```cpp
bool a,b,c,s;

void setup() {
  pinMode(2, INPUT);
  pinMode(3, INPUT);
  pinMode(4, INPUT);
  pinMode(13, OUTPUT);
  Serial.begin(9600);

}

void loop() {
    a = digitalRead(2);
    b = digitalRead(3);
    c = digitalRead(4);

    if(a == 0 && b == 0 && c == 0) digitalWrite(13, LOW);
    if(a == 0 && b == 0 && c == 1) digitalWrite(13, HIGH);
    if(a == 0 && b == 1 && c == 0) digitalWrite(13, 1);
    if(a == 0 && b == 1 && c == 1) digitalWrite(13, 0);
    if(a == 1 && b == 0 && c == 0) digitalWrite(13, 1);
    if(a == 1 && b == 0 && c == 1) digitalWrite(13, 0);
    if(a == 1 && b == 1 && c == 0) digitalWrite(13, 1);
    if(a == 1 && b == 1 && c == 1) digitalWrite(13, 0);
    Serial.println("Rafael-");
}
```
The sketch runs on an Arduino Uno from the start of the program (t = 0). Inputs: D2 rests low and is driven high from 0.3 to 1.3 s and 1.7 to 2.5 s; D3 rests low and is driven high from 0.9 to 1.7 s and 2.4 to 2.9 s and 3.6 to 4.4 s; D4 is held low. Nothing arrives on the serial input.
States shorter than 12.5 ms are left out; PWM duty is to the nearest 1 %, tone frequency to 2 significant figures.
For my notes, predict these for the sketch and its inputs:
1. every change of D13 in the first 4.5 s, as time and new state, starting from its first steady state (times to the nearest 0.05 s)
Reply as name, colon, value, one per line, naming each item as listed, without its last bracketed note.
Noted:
every change of D13 in the first 4.5 s, as time and new state, starting from its first steady state: 0 s low; 0.3 s high; 2.9 s low; 3.6 s high; 4.4 s low
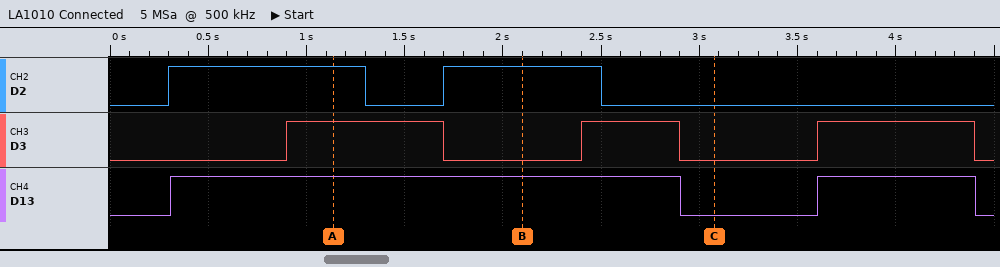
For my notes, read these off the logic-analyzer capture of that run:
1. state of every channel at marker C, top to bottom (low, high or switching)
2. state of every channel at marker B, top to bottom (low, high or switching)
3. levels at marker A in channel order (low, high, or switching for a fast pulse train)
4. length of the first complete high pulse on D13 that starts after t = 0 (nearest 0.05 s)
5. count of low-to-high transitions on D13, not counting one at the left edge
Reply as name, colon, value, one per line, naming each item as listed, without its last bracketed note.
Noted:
state of every channel at marker C, top to bottom: D2 low, D3 low, D13 low
state of every channel at marker B, top to bottom: D2 high, D3 low, D13 high
levels at marker A in channel order: D2 high, D3 high, D13 high
length of the first complete high pulse on D13 that starts after t = 0: 2.60 s
count of low-to-high transitions on D13, not counting one at the left edge: 2
